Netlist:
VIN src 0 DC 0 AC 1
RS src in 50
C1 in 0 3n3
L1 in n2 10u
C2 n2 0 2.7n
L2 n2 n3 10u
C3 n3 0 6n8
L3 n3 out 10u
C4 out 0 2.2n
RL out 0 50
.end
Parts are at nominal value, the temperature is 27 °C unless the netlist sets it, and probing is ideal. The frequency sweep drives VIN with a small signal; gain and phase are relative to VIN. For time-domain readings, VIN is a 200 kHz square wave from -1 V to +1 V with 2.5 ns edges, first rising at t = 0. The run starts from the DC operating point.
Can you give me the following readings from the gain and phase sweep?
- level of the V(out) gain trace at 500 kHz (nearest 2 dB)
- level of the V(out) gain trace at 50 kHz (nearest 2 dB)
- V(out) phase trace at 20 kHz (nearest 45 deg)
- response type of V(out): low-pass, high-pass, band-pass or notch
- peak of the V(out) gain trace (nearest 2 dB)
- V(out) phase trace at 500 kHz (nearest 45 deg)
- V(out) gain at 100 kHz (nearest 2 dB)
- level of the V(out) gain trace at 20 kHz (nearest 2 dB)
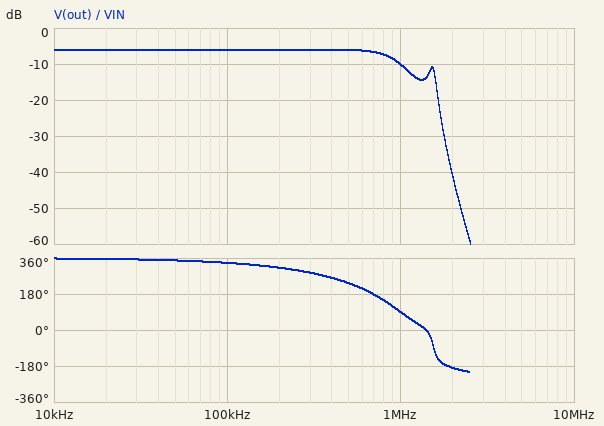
-6 dB
-6 dB
360 deg
low-pass
-6 dB
225 deg
-6 dB
-6 dB
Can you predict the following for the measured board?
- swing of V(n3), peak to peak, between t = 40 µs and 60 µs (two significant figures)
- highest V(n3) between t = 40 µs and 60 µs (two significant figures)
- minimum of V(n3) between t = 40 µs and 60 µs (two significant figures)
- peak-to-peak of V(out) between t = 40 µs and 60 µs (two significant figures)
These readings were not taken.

1.2 V
590 mV
-590 mV
1.2 V
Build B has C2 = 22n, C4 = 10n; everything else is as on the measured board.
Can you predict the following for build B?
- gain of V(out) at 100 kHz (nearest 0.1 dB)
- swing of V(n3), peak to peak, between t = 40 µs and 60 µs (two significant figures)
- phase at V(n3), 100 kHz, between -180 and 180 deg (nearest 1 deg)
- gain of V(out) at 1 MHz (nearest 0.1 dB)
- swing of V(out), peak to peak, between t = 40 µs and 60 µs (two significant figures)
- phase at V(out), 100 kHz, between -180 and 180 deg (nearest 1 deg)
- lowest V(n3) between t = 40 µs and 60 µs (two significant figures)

-6.8 dB
1.1 V
-38 deg
-15.7 dB
960 mV
-46 deg
-560 mV
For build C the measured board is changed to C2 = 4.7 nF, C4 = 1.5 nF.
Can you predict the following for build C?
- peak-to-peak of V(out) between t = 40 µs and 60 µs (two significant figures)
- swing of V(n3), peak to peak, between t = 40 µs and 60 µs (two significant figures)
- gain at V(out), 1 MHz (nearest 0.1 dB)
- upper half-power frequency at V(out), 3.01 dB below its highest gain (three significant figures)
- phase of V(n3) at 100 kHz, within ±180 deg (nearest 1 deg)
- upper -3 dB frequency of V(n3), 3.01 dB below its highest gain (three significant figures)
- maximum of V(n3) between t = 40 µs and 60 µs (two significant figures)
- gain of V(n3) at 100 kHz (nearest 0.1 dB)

1.3 V
1.4 V
-8.2 dB
1.27 MHz
-18 deg
1.30 MHz
690 mV
-6.0 dB
